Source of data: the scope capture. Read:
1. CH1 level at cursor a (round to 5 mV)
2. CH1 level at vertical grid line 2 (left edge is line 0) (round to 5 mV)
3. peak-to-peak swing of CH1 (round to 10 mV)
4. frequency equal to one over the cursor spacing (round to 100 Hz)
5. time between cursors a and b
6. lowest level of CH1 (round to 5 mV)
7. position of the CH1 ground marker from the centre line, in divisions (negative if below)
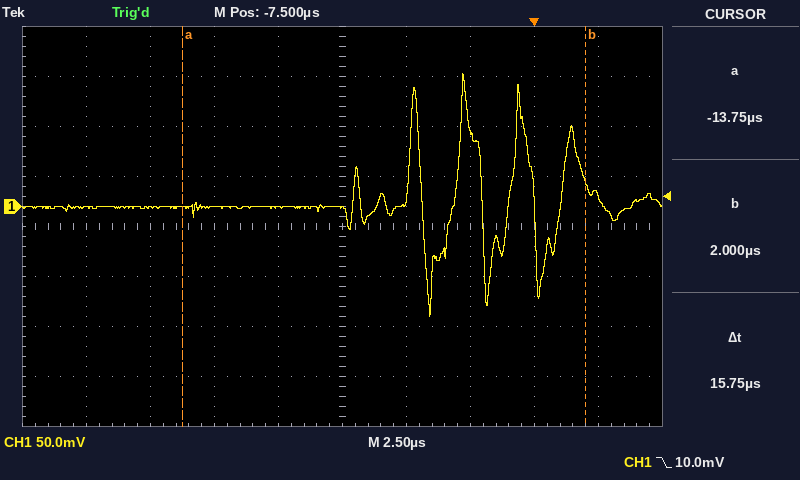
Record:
0 mV
0 mV
240 mV
63.5 kHz
15.75 µs
-110 mV
+0.4 div
